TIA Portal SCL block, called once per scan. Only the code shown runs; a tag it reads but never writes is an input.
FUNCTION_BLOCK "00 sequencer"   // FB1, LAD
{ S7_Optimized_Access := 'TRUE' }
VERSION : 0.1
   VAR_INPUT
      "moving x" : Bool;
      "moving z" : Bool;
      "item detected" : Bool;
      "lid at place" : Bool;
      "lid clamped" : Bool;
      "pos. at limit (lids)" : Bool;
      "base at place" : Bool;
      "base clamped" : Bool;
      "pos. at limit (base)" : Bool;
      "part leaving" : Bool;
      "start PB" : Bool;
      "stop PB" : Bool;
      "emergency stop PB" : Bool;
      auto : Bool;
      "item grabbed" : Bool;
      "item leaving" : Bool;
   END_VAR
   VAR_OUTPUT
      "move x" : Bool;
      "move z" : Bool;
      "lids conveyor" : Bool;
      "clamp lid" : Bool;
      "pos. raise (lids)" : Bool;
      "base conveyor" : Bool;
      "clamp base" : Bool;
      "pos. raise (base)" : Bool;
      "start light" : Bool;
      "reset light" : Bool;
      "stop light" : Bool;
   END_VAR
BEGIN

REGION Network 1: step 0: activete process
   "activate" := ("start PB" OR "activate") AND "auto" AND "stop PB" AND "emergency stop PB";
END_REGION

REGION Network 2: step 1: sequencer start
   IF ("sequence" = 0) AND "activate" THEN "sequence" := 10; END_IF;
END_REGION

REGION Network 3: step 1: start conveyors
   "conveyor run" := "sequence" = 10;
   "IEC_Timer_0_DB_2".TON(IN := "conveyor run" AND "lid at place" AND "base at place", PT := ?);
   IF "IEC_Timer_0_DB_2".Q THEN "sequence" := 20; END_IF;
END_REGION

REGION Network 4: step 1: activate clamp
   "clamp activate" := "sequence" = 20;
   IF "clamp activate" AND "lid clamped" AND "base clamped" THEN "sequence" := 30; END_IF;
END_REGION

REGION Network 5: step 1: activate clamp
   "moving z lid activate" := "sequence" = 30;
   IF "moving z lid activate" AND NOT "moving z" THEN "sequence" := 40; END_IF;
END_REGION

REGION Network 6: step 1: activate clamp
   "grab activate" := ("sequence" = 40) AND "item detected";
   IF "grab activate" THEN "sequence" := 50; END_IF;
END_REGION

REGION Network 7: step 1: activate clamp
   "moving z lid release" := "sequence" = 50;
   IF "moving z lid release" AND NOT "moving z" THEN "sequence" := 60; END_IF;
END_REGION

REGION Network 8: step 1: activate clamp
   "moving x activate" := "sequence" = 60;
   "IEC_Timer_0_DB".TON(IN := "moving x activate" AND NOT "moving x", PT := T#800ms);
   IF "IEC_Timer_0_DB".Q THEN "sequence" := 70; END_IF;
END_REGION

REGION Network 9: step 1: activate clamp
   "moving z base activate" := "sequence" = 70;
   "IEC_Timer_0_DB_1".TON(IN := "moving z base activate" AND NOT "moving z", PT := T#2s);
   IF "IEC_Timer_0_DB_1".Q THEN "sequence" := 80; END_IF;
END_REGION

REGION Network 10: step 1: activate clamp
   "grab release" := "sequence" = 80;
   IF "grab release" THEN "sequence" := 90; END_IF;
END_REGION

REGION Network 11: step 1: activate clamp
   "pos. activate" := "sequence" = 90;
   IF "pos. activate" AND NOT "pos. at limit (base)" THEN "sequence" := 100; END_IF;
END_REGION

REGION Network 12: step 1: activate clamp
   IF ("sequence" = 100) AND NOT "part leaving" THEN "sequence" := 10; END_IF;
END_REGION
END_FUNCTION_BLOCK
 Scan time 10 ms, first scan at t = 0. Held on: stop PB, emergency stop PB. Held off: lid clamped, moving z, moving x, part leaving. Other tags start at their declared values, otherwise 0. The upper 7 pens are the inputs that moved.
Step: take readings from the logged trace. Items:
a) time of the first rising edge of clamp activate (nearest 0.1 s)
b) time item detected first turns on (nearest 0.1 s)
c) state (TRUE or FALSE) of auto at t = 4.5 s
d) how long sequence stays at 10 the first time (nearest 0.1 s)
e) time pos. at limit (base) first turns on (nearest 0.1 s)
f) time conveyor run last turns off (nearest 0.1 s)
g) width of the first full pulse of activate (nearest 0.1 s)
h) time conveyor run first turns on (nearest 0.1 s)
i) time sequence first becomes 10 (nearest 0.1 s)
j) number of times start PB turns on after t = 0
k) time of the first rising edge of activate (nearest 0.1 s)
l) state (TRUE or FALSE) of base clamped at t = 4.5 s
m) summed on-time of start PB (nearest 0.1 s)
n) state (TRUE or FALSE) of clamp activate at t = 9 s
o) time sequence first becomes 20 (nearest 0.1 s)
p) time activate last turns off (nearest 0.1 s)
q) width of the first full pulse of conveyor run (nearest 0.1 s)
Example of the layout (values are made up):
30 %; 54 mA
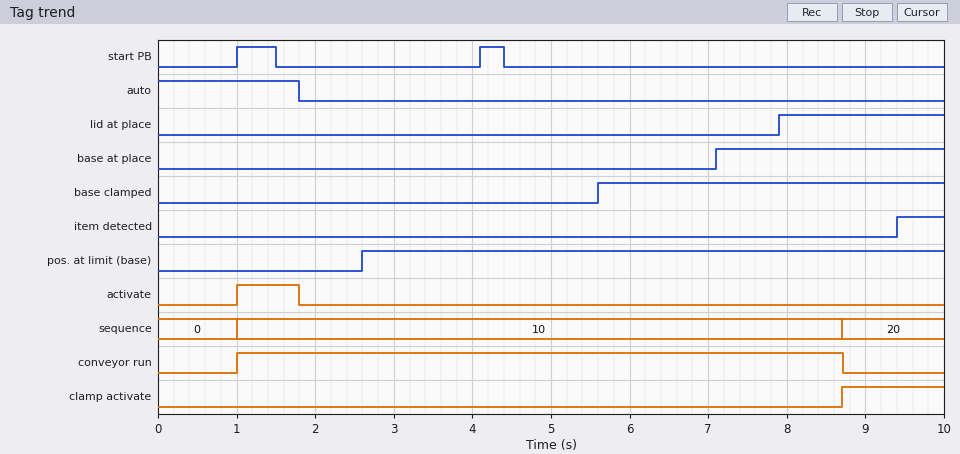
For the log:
8.7 s; 9.4 s; FALSE; 7.7 s; 2.6 s; 8.7 s; 0.8 s; 1.0 s; 1.0 s; 2; 1.0 s; FALSE; 0.8 s; TRUE; 8.7 s; 1.8 s; 7.7 s
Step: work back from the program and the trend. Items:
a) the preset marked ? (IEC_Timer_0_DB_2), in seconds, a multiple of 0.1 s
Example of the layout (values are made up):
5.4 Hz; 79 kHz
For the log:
0.8 s
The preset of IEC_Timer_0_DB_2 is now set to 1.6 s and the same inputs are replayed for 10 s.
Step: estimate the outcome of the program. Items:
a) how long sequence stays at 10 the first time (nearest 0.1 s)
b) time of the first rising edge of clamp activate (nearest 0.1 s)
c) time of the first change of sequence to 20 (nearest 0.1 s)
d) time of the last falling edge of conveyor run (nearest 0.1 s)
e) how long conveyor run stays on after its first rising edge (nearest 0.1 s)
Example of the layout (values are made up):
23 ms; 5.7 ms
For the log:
8.5 s; 9.5 s; 9.5 s; 9.5 s; 8.5 s
